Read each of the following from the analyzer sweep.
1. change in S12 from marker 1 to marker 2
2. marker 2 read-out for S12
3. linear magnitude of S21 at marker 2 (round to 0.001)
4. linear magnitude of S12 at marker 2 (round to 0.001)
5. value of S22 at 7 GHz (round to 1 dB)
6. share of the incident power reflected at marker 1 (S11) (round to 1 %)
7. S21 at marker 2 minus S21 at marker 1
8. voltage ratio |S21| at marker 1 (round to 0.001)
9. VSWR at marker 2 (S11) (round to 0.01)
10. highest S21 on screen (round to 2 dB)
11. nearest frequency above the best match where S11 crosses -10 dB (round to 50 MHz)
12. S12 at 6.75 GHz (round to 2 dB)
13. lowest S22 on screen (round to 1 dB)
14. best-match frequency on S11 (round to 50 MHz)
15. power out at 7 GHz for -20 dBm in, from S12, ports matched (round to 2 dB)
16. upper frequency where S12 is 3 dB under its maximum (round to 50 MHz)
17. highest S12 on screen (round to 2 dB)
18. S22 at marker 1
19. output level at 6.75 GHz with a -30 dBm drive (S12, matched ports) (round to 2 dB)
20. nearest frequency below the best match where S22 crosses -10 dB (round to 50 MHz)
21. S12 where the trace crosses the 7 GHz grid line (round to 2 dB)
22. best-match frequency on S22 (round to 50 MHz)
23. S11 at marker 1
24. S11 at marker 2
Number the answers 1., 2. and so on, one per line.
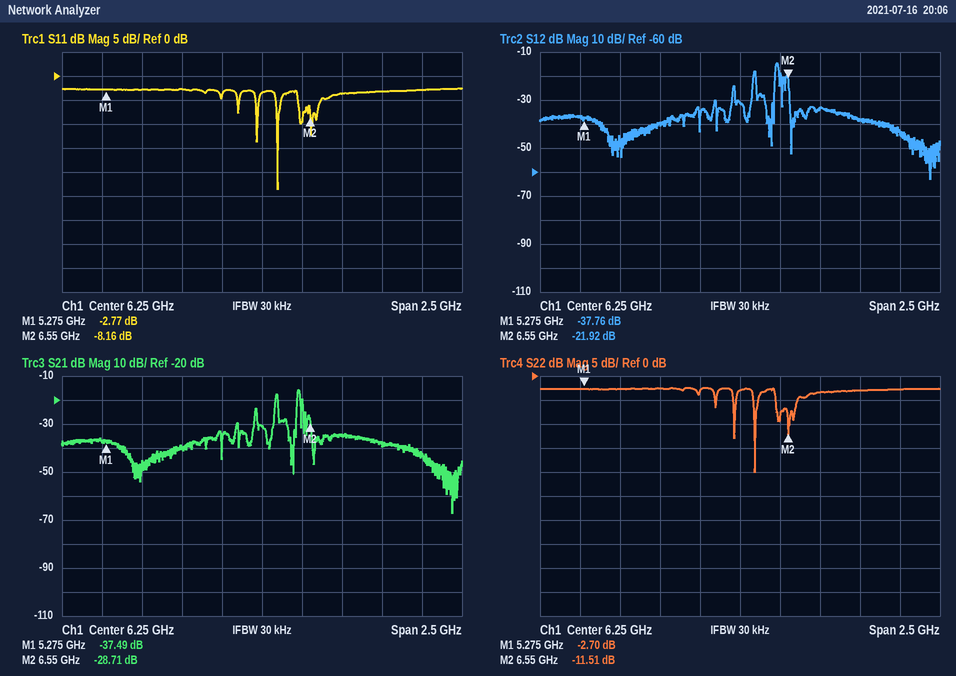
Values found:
1. 15.84 dB
2. -21.92 dB
3. 0.037
4. 0.080
5. -3 dB
6. 53 %
7. 8.78 dB
8. 0.013
9. 2.28
10. -16 dB
11. 6.35 GHz
12. -34 dB
13. -20 dB
14. 6.35 GHz
15. -58 dBm
16. 6.50 GHz
17. -14 dB
18. -2.70 dB
19. -64 dBm
20. 6.35 GHz
21. -38 dB
22. 6.35 GHz
23. -2.77 dB
24. -8.16 dB
